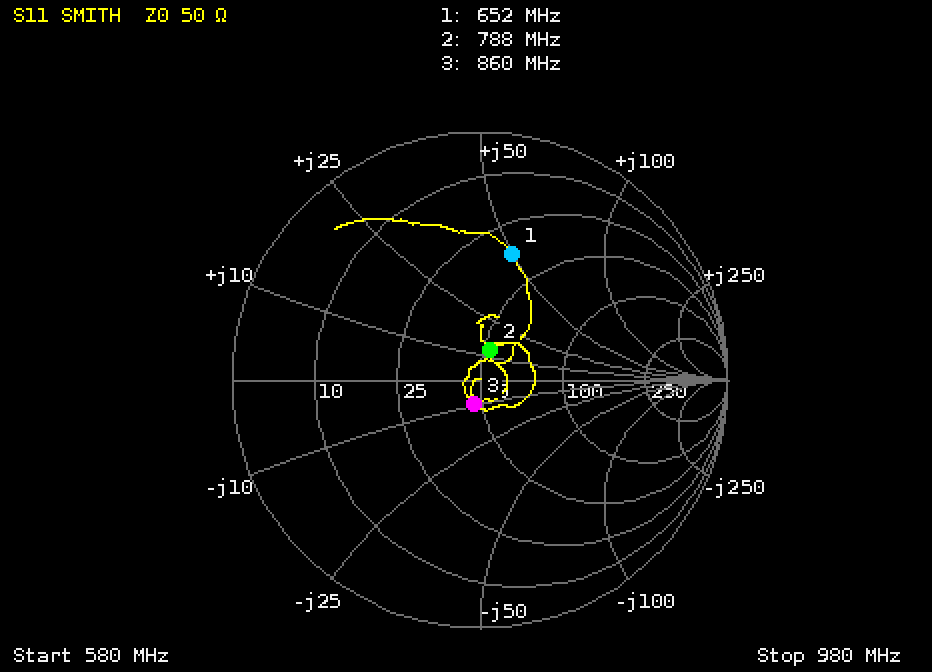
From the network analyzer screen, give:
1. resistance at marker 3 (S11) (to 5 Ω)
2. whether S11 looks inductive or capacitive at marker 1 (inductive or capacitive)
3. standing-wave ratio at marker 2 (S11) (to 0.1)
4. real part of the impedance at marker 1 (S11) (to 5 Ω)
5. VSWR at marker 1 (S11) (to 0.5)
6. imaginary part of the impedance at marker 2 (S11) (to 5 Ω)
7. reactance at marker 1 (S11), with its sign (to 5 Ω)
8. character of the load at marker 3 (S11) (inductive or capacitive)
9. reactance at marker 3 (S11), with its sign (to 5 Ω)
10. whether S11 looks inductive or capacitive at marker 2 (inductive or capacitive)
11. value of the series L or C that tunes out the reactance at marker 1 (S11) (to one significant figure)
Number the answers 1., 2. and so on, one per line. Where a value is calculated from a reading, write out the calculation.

1. 45 Ω
2. inductive
3. 1.3
4. 35 Ω
5. 3.0
6. +15 Ω
7. +50 Ω
8. capacitive
9. -10 Ω
10. inductive
11. C = 1/(2π × 652 MHz × 50 Ω) ≈ 5 pF
